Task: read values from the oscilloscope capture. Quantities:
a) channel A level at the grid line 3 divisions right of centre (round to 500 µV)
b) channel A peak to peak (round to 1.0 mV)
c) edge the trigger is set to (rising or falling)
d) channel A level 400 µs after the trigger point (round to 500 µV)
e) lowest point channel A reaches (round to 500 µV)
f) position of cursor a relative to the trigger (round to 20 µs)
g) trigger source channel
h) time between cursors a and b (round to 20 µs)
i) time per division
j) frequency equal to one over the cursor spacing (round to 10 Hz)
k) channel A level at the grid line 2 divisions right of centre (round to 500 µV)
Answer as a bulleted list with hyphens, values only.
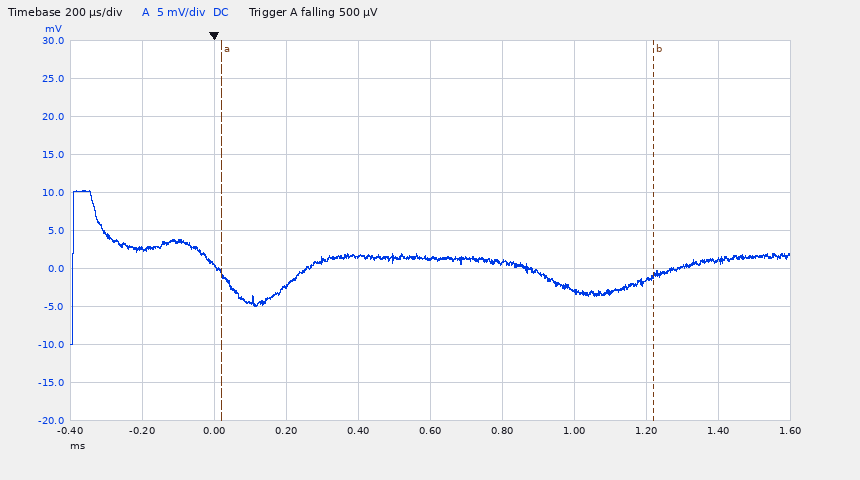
- -1.5 mV
- 20.0 mV
- falling
- 1.5 mV
- -10.0 mV
- +20 µs
- channel A
- 1.20 ms
- 200 µs
- 830 Hz
- -3.0 mV
